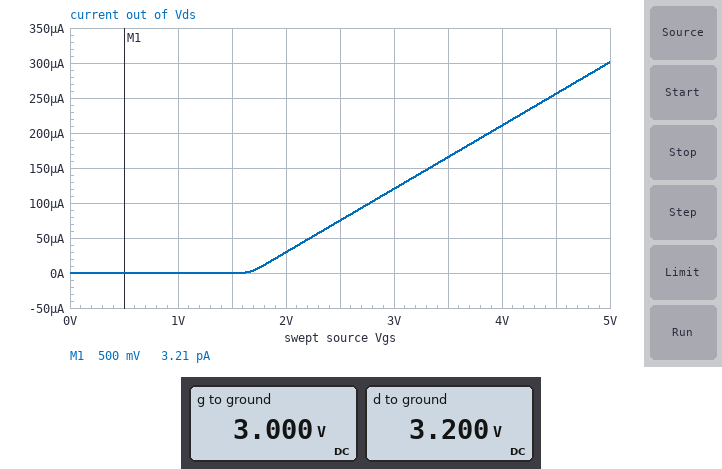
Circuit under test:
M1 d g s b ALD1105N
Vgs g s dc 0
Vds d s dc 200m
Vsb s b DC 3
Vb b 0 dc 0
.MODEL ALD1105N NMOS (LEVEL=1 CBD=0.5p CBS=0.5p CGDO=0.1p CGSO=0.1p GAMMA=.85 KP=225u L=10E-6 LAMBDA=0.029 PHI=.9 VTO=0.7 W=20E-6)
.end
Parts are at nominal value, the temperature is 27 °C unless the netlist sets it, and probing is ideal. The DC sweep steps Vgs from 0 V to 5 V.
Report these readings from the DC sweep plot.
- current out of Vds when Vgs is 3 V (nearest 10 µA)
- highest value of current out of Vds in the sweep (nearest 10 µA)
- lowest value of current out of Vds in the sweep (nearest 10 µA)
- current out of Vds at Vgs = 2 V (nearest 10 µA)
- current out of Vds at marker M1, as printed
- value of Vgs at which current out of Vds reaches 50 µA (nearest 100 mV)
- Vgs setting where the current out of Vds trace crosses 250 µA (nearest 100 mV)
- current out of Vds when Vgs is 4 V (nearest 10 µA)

120 µA
300 µA
0 A
30 µA
3.21 pA
2.2 V
4.4 V
210 µA
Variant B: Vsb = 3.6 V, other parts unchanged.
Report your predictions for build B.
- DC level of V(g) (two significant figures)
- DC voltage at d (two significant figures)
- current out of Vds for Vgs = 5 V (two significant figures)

3.6 V
3.8 V
290 µA
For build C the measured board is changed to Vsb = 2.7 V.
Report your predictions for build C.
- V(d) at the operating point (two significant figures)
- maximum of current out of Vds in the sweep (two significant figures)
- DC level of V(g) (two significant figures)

2.9 V
310 µA
2.7 V
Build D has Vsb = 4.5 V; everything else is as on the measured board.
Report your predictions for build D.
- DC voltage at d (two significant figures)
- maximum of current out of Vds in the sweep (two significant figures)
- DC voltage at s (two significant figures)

4.7 V
270 µA
4.5 V
